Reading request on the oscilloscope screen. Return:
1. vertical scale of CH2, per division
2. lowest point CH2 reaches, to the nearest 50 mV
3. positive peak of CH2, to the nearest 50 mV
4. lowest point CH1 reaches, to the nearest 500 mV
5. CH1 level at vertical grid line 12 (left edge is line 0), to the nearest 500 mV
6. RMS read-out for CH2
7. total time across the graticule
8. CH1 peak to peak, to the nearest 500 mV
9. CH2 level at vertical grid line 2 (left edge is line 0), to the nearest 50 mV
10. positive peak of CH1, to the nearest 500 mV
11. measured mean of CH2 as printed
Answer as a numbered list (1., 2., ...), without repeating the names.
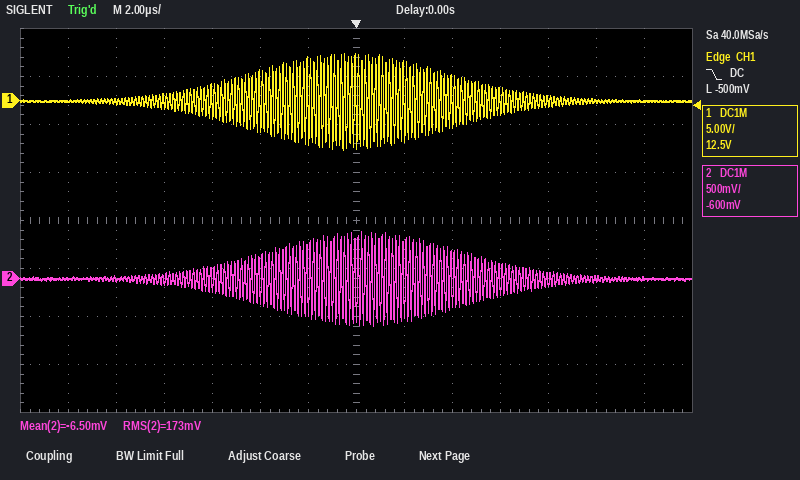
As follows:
1. 500 mV
2. -500 mV
3. 500 mV
4. -5.0 V
5. 0.0 V
6. 173 mV
7. 28 µs
8. 10.0 V
9. 0 mV
10. 5.0 V
11. -6.50 mV
